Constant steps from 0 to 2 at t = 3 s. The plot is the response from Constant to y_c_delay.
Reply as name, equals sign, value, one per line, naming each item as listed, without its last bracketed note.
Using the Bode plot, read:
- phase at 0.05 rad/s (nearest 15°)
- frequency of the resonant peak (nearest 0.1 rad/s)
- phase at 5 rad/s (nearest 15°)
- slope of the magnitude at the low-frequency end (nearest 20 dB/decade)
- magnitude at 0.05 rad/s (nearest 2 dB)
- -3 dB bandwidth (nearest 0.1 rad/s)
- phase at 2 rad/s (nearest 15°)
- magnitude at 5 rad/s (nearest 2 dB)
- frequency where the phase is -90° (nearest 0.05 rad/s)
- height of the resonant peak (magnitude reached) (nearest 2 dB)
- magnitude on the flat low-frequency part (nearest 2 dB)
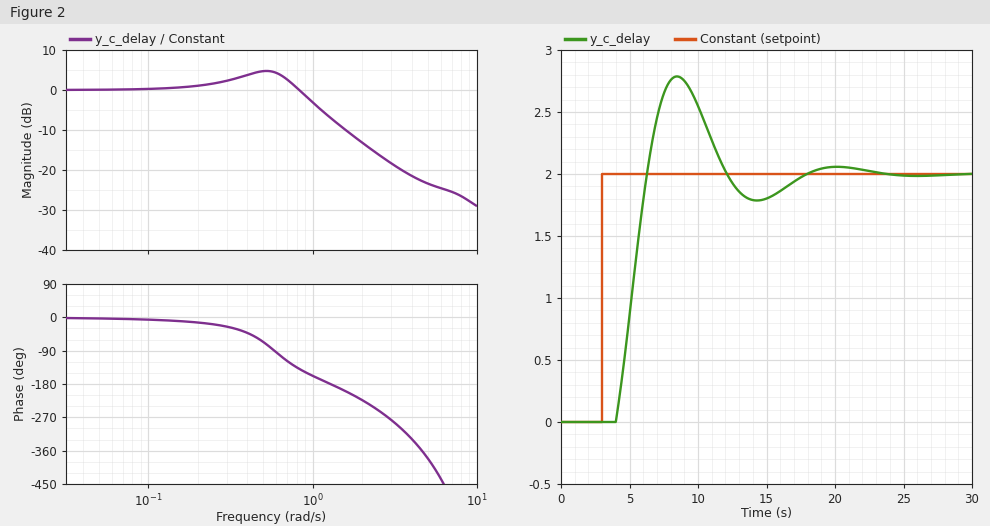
phase at 0.05 rad/s = 0°
frequency of the resonant peak = 0.5 rad/s
phase at 5 rad/s = -375°
slope of the magnitude at the low-frequency end = 0 dB/decade
magnitude at 0.05 rad/s = 0 dB
-3 dB bandwidth = 1.0 rad/s
phase at 2 rad/s = -225°
magnitude at 5 rad/s = -24 dB
frequency where the phase is -90° = 0.60 rad/s
height of the resonant peak (magnitude reached) = 4 dB
magnitude on the flat low-frequency part = 0 dB
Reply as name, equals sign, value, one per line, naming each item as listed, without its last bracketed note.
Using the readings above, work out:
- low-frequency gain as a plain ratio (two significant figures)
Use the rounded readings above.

low-frequency gain as a plain ratio = 1.0
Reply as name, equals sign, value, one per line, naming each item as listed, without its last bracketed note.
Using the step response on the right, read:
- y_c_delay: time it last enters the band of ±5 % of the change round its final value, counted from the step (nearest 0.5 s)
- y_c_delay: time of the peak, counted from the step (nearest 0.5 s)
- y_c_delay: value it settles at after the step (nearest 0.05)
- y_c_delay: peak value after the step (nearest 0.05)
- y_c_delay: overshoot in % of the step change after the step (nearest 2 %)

y_c_delay: time it last enters the band of ±5 % of the change round its final value, counted from the step = 13.5 s
y_c_delay: time of the peak, counted from the step = 5.5 s
y_c_delay: value it settles at after the step = 2.00
y_c_delay: peak value after the step = 2.80
y_c_delay: overshoot in % of the step change after the step = 40 %
